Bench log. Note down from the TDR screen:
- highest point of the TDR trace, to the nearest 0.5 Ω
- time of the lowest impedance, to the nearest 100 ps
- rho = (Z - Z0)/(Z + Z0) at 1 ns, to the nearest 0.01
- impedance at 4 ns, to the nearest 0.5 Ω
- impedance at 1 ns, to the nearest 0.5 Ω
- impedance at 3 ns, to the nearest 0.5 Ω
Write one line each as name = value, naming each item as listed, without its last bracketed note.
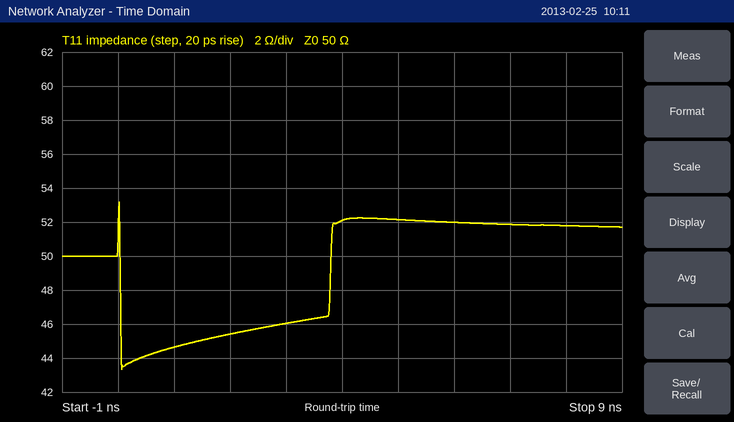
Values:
highest point of the TDR trace, to the nearest 0.5 Ω = 53.0 Ω
time of the lowest impedance, to the nearest 100 ps = 100 ps
rho = (Z - Z0)/(Z + Z0) at 1 ns, to the nearest 0.01 = -0.06
impedance at 4 ns, to the nearest 0.5 Ω = 52.0 Ω
impedance at 1 ns, to the nearest 0.5 Ω = 44.5 Ω
impedance at 3 ns, to the nearest 0.5 Ω = 46.0 Ω
